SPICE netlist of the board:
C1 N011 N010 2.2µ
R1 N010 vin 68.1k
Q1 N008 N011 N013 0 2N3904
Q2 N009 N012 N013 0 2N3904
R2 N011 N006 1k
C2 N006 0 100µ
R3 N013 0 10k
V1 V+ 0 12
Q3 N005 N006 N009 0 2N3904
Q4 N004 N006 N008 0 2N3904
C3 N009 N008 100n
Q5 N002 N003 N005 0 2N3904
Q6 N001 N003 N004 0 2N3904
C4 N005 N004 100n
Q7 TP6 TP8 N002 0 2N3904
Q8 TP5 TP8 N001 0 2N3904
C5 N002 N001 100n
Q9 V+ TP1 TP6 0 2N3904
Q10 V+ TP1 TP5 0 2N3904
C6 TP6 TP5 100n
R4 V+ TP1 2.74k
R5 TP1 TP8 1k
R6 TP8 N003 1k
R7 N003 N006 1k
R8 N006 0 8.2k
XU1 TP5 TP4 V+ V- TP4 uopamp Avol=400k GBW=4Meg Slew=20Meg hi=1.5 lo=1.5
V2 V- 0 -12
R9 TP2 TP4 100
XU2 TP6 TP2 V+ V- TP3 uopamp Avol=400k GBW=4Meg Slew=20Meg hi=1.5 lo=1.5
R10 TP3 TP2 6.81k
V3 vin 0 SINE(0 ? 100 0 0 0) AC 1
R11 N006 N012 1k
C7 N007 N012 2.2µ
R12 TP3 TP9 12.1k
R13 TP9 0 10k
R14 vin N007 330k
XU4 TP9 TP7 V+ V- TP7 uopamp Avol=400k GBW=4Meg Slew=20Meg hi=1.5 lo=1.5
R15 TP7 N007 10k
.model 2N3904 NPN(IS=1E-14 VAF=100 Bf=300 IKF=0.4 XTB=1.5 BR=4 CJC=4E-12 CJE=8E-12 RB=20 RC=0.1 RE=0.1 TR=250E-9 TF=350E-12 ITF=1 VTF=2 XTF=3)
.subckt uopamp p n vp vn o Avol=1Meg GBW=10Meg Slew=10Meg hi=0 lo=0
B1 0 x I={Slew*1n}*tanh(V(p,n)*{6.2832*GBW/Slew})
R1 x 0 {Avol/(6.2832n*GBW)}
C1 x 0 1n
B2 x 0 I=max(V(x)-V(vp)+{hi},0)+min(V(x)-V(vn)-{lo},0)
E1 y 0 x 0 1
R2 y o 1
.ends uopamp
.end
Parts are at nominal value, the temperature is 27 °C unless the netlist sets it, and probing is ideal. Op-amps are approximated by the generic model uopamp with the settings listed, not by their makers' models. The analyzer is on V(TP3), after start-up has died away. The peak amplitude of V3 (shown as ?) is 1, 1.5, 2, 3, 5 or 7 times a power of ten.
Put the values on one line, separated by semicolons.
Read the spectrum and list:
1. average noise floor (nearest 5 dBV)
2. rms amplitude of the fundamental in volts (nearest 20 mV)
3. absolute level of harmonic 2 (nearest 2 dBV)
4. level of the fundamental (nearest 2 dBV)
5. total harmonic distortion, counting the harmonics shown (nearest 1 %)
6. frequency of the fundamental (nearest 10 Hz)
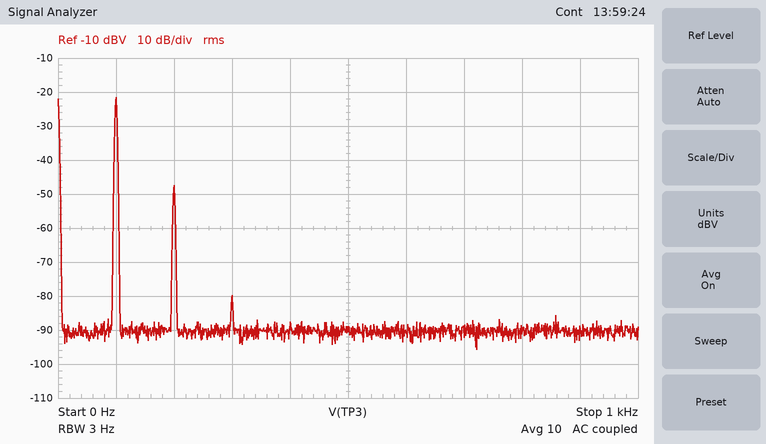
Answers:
-90 dBV; 80 mV; -48 dBV; -22 dBV; 5 %; 100 Hz
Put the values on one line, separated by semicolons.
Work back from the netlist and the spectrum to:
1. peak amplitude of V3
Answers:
1 V
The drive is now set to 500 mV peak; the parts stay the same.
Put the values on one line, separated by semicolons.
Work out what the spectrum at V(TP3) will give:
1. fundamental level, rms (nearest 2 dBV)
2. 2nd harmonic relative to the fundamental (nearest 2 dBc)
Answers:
-28 dBV; -32 dBc
